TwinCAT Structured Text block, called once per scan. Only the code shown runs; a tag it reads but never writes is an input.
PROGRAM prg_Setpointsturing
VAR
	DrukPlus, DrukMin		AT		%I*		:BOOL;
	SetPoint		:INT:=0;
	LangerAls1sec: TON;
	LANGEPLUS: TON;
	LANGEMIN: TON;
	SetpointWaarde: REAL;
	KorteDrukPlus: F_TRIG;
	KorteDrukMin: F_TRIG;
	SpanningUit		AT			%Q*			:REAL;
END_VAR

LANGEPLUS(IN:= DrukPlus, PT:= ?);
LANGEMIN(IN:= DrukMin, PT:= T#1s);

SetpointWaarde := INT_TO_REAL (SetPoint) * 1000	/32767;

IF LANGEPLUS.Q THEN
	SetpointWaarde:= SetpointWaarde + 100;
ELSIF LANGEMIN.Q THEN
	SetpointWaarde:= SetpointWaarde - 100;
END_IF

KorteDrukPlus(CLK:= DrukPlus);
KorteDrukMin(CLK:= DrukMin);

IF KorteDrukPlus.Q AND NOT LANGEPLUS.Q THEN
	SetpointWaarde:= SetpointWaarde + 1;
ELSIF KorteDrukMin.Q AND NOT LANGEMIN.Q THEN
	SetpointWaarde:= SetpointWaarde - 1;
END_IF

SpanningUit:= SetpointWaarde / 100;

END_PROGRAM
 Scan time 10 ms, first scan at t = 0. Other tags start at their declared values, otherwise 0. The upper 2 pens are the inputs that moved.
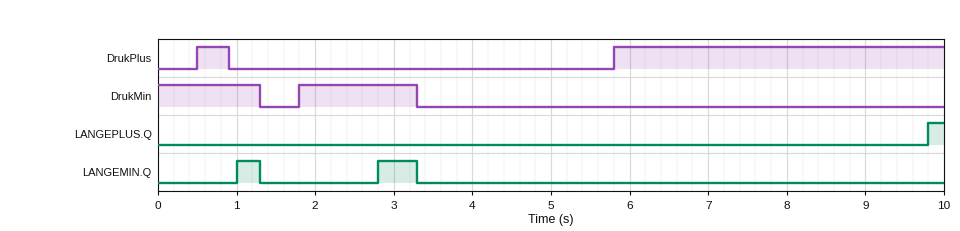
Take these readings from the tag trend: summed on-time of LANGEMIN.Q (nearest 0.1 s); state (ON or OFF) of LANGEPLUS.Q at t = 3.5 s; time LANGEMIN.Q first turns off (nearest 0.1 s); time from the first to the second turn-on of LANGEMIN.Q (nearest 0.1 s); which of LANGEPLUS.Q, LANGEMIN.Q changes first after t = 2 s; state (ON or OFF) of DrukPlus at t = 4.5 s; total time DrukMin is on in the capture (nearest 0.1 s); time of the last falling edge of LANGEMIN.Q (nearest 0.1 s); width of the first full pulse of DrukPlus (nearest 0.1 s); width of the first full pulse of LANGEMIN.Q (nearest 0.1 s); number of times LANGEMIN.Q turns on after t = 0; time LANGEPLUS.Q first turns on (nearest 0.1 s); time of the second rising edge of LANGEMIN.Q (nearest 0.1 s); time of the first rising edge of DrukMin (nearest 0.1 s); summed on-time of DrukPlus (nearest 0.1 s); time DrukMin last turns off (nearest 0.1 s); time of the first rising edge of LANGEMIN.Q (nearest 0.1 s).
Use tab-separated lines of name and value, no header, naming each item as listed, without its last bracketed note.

summed on-time of LANGEMIN.Q	0.8 s
state (ON or OFF) of LANGEPLUS.Q at t = 3.5 s	OFF
time LANGEMIN.Q first turns off	1.3 s
time from the first to the second turn-on of LANGEMIN.Q	1.8 s
which of LANGEPLUS.Q, LANGEMIN.Q changes first after t = 2 s	LANGEMIN.Q
state (ON or OFF) of DrukPlus at t = 4.5 s	OFF
total time DrukMin is on in the capture	2.8 s
time of the last falling edge of LANGEMIN.Q	3.3 s
width of the first full pulse of DrukPlus	0.4 s
width of the first full pulse of LANGEMIN.Q	0.3 s
number of times LANGEMIN.Q turns on after t = 0	2
time LANGEPLUS.Q first turns on	9.8 s
time of the second rising edge of LANGEMIN.Q	2.8 s
time of the first rising edge of DrukMin	1.8 s
summed on-time of DrukPlus	4.6 s
time DrukMin last turns off	3.3 s
time of the first rising edge of LANGEMIN.Q	1.0 s
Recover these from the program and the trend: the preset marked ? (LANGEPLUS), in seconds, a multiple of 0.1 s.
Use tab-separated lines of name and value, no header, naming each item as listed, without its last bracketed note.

the preset marked ? (LANGEPLUS), in seconds, a multiple of 0.1 s	4.0 s
